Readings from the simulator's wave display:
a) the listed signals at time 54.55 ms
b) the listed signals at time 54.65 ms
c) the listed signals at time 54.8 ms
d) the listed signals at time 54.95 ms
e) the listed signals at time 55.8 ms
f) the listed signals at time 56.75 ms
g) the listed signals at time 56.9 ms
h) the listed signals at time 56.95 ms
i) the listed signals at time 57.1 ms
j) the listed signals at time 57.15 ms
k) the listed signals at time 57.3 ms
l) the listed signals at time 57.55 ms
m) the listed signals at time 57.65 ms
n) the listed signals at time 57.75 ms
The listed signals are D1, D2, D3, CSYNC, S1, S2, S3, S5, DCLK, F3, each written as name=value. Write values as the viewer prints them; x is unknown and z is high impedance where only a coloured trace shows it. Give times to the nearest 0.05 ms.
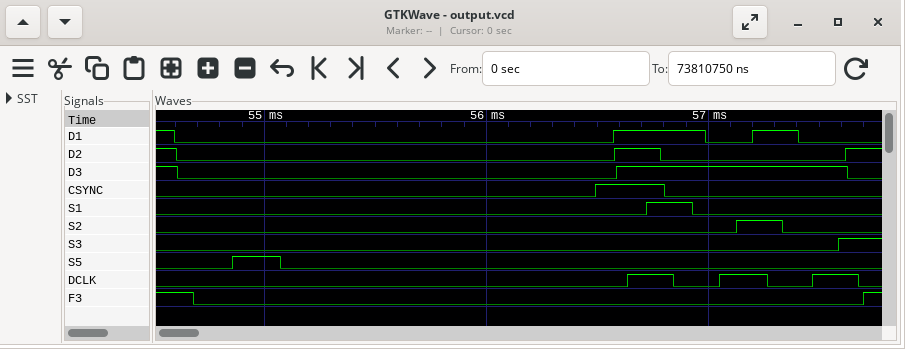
D1=1, D2=1, D3=1, CSYNC=0, S1=0, S2=0, S3=0, S5=0, DCLK=0, F3=1
D1=0, D2=0, D3=0, CSYNC=0, S1=0, S2=0, S3=0, S5=0, DCLK=0, F3=1
D1=0, D2=0, D3=0, CSYNC=0, S1=0, S2=0, S3=0, S5=0, DCLK=0, F3=0
D1=0, D2=0, D3=0, CSYNC=0, S1=0, S2=0, S3=0, S5=1, DCLK=0, F3=0
D1=0, D2=0, D3=0, CSYNC=0, S1=0, S2=0, S3=0, S5=0, DCLK=0, F3=0
D1=1, D2=1, D3=1, CSYNC=1, S1=1, S2=0, S3=0, S5=0, DCLK=1, F3=0
D1=1, D2=0, D3=1, CSYNC=0, S1=1, S2=0, S3=0, S5=0, DCLK=0, F3=0
D1=1, D2=0, D3=1, CSYNC=0, S1=0, S2=0, S3=0, S5=0, DCLK=0, F3=0
D1=0, D2=0, D3=1, CSYNC=0, S1=0, S2=0, S3=0, S5=0, DCLK=1, F3=0
D1=0, D2=0, D3=1, CSYNC=0, S1=0, S2=1, S3=0, S5=0, DCLK=1, F3=0
D1=1, D2=0, D3=1, CSYNC=0, S1=0, S2=1, S3=0, S5=0, DCLK=0, F3=0
D1=0, D2=0, D3=1, CSYNC=0, S1=0, S2=0, S3=0, S5=0, DCLK=1, F3=0
D1=0, D2=1, D3=0, CSYNC=0, S1=0, S2=0, S3=1, S5=0, DCLK=1, F3=0
D1=0, D2=1, D3=0, CSYNC=0, S1=0, S2=0, S3=1, S5=0, DCLK=0, F3=1
